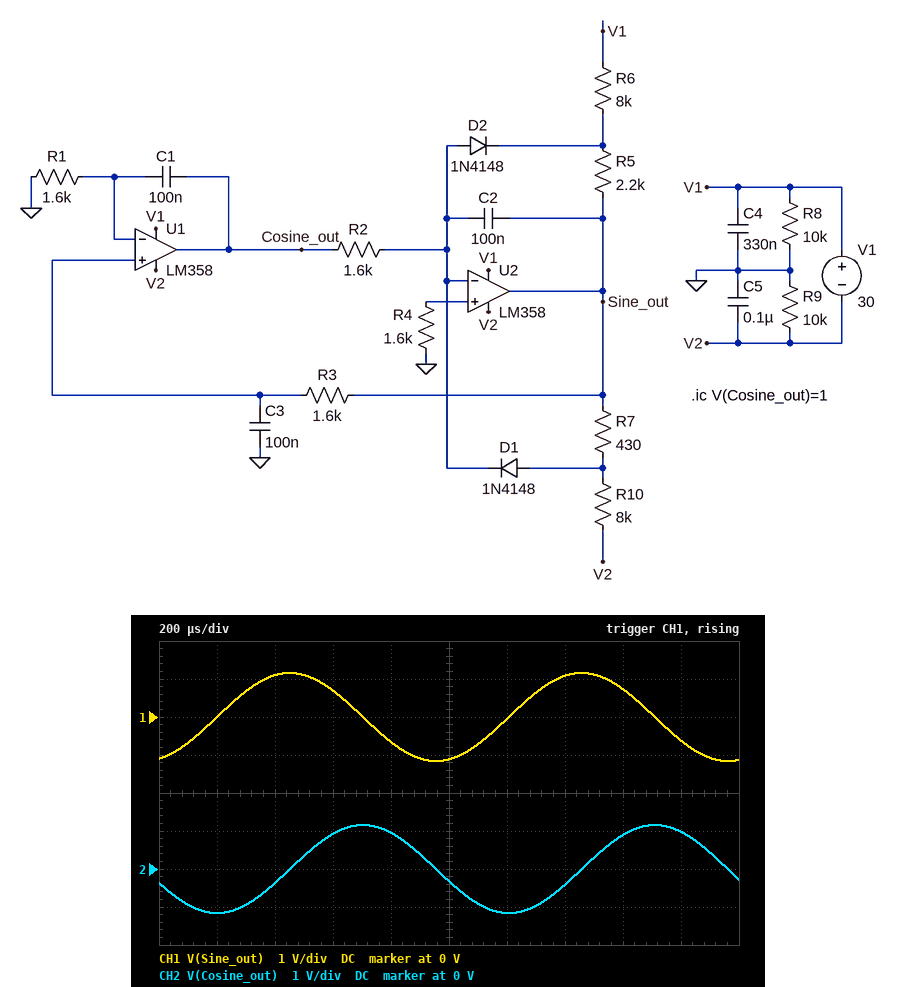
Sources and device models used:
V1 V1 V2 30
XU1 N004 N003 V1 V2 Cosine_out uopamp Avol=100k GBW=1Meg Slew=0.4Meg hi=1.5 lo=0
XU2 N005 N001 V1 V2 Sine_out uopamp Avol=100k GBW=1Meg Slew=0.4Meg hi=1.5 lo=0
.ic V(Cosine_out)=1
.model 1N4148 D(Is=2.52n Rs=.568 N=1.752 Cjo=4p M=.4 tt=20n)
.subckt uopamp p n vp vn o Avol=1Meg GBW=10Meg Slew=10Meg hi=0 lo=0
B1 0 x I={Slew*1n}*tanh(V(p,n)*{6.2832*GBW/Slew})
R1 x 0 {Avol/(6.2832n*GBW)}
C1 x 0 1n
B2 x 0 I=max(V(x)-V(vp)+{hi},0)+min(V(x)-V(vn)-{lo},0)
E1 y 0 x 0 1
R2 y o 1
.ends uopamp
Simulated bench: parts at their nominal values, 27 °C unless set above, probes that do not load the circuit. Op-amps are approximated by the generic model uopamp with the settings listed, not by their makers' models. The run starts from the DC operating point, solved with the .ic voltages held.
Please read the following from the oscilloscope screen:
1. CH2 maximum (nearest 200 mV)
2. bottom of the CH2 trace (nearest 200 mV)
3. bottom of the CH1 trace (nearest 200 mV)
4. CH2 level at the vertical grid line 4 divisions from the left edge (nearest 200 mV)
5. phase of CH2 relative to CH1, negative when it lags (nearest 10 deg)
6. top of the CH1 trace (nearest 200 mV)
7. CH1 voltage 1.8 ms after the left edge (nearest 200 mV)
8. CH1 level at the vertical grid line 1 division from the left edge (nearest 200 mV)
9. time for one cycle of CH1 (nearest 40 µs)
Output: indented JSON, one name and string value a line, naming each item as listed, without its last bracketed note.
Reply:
{
  "CH2 maximum": "1.2 V",
  "bottom of the CH2 trace": "-1.2 V",
  "bottom of the CH1 trace": "-1.2 V",
  "CH2 level at the vertical grid line 4 divisions from the left edge": "1.0 V",
  "phase of CH2 relative to CH1, negative when it lags": "-90 deg",
  "top of the CH1 trace": "1.2 V",
  "CH1 voltage 1.8 ms after the left edge": "-600 mV",
  "CH1 level at the vertical grid line 1 division from the left edge": "0 V",
  "time for one cycle of CH1": "1.00 ms"
}
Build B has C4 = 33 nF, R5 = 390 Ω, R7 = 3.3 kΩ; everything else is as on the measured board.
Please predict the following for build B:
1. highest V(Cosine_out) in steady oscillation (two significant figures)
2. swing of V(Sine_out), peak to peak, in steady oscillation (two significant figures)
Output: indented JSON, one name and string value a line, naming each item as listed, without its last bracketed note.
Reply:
{
  "highest V(Cosine_out) in steady oscillation": "1.1 V",
  "swing of V(Sine_out), peak to peak, in steady oscillation": "2.1 V"
}
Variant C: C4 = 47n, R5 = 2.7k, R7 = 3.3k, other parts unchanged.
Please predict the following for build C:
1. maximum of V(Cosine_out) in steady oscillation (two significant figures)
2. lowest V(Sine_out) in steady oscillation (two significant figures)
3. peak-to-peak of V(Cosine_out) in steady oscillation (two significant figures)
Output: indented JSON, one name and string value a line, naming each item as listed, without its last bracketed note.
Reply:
{
  "maximum of V(Cosine_out) in steady oscillation": "5.6 V",
  "lowest V(Sine_out) in steady oscillation": "-5.6 V",
  "peak-to-peak of V(Cosine_out) in steady oscillation": "11 V"
}
